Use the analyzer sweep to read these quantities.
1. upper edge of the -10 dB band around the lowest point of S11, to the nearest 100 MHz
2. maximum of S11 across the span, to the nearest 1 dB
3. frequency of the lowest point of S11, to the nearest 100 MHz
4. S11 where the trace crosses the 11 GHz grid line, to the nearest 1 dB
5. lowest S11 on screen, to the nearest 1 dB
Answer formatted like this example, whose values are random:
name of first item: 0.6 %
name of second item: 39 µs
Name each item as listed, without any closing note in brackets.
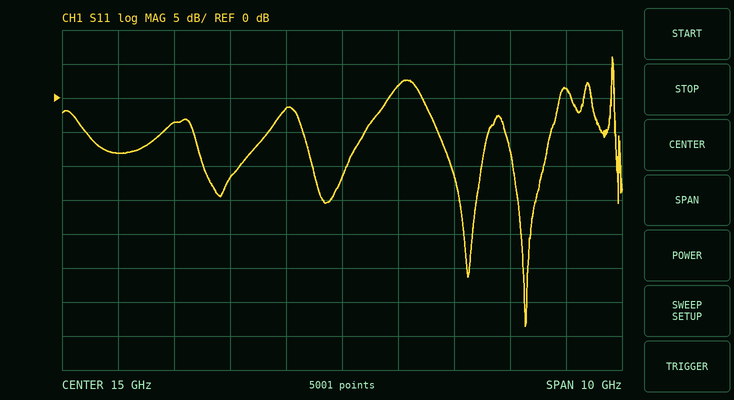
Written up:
upper edge of the -10 dB band around the lowest point of S11, to the nearest 100 MHz: 18.6 GHz
maximum of S11 across the span, to the nearest 1 dB: 6 dB
frequency of the lowest point of S11, to the nearest 100 MHz: 18.3 GHz
S11 where the trace crosses the 11 GHz grid line, to the nearest 1 dB: -8 dB
lowest S11 on screen, to the nearest 1 dB: -34 dB
